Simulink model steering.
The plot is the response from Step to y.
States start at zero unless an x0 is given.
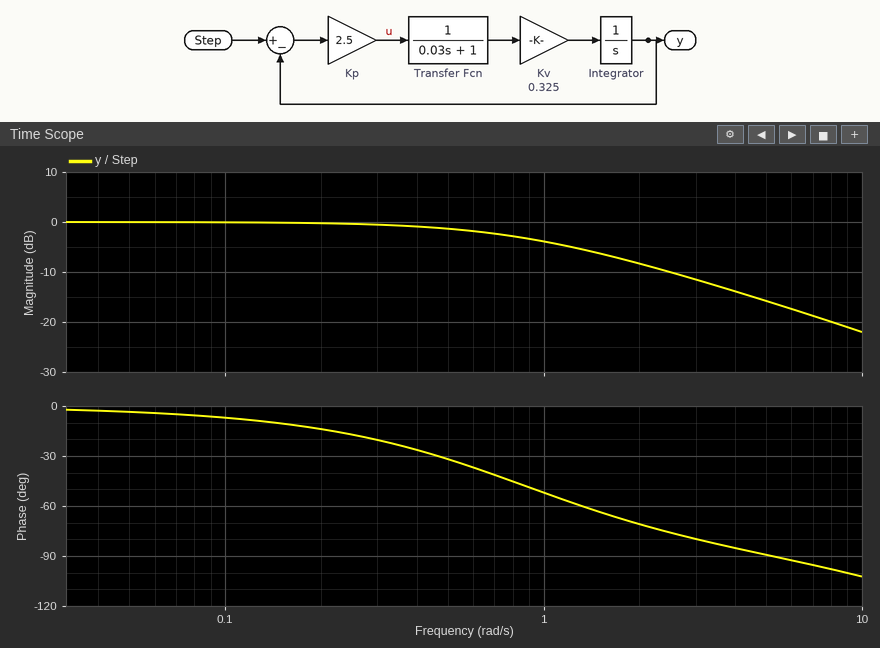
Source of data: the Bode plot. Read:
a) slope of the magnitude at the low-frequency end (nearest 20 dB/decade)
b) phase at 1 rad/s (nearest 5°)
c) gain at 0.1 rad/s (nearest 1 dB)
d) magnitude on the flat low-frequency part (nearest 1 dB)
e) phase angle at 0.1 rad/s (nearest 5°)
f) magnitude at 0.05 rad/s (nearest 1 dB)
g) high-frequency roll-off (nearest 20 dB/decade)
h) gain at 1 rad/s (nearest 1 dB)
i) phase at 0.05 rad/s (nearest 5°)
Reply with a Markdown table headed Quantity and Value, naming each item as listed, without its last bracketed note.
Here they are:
| Quantity | Value |
|---|---|
| slope of the magnitude at the low-frequency end | 0 dB/decade |
| phase at 1 rad/s | -50° |
| gain at 0.1 rad/s | 0 dB |
| magnitude on the flat low-frequency part | 0 dB |
| phase angle at 0.1 rad/s | -5° |
| magnitude at 0.05 rad/s | 0 dB |
| high-frequency roll-off | -20 dB/decade |
| gain at 1 rad/s | -4 dB |
| phase at 0.05 rad/s | -5° |
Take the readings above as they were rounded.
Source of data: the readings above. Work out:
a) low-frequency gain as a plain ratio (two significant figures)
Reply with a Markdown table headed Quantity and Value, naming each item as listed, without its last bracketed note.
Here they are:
| Quantity | Value |
|---|---|
| low-frequency gain as a plain ratio | 1.0 |
